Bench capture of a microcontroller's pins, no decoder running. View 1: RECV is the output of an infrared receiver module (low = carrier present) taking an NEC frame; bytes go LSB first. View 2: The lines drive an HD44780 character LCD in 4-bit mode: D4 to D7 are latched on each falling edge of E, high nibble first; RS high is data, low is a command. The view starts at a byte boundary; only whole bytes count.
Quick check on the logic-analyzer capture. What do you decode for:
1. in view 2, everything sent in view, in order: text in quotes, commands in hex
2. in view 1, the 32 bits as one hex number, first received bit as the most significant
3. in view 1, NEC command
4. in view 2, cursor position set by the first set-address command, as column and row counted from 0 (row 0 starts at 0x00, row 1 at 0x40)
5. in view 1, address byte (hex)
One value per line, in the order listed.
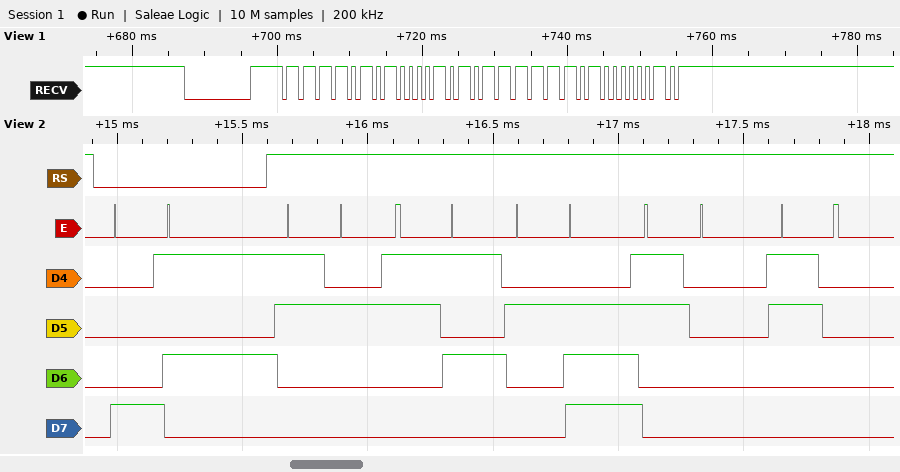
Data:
0x85 "25.00"
0xF50AFD02
0xBF
column 5, row 0
0xAF
